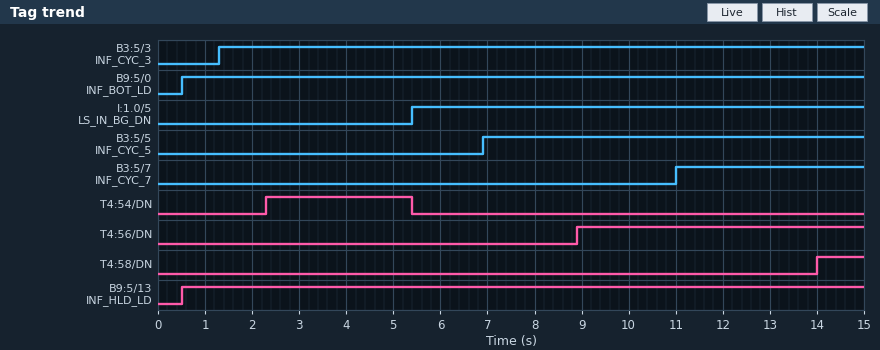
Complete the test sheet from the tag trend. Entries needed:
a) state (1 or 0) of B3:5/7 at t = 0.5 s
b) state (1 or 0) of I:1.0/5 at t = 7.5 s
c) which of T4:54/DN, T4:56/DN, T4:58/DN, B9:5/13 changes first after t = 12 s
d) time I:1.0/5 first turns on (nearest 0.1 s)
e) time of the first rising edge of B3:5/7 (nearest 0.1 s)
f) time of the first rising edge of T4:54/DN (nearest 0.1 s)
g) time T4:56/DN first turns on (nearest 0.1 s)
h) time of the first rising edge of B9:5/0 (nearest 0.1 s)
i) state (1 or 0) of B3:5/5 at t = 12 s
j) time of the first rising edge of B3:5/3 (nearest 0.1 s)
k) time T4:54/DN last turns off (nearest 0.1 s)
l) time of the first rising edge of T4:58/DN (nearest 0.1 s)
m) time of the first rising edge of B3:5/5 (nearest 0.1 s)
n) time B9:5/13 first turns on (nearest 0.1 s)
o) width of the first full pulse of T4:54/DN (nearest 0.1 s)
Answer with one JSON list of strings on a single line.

["0", "1", "T4:58/DN", "5.4 s", "11.0 s", "2.3 s", "8.9 s", "0.5 s", "1", "1.3 s", "5.4 s", "14.0 s", "6.9 s", "0.5 s", "3.1 s"]
